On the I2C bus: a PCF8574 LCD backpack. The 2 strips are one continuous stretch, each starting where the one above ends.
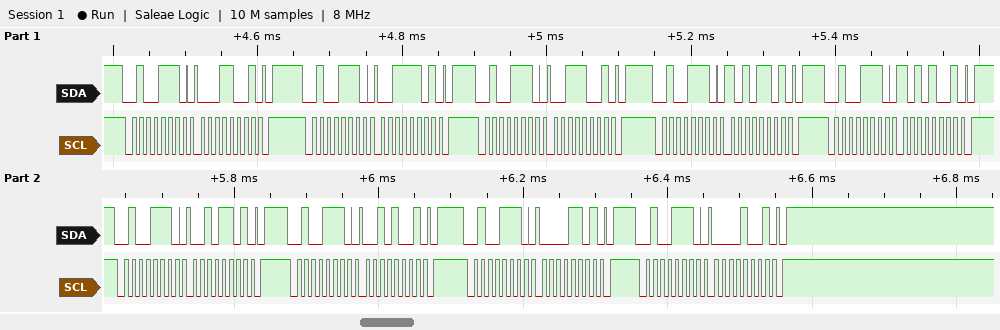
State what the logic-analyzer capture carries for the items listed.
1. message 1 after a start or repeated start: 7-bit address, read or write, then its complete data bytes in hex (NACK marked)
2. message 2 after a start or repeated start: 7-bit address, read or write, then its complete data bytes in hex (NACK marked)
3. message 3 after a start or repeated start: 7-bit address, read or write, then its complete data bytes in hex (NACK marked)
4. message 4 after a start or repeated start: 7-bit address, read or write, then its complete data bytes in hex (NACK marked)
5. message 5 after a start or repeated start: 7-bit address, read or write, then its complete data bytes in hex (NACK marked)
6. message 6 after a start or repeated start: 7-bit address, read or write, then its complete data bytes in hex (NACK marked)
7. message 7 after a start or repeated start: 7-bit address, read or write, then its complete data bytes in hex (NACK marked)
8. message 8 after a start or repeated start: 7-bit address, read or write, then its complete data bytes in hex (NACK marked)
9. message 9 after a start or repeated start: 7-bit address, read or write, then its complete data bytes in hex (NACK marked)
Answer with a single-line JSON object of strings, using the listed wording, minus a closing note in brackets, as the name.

{"message 1 after a start or repeated start: 7-bit address, read or write, then its complete data bytes in hex": "0x27 write: 19", "message 2 after a start or repeated start: 7-bit address, read or write, then its complete data bytes in hex": "0x27 write: 3D", "message 3 after a start or repeated start: 7-bit address, read or write, then its complete data bytes in hex": "0x27 write: 39", "message 4 after a start or repeated start: 7-bit address, read or write, then its complete data bytes in hex": "0x27 write: AD", "message 5 after a start or repeated start: 7-bit address, read or write, then its complete data bytes in hex": "0x27 write: A9", "message 6 after a start or repeated start: 7-bit address, read or write, then its complete data bytes in hex": "0x27 write: 2D", "message 7 after a start or repeated start: 7-bit address, read or write, then its complete data bytes in hex": "0x27 write: 29", "message 8 after a start or repeated start: 7-bit address, read or write, then its complete data bytes in hex": "0x27 write: 0D", "message 9 after a start or repeated start: 7-bit address, read or write, then its complete data bytes in hex": "0x27 write: 09"}
